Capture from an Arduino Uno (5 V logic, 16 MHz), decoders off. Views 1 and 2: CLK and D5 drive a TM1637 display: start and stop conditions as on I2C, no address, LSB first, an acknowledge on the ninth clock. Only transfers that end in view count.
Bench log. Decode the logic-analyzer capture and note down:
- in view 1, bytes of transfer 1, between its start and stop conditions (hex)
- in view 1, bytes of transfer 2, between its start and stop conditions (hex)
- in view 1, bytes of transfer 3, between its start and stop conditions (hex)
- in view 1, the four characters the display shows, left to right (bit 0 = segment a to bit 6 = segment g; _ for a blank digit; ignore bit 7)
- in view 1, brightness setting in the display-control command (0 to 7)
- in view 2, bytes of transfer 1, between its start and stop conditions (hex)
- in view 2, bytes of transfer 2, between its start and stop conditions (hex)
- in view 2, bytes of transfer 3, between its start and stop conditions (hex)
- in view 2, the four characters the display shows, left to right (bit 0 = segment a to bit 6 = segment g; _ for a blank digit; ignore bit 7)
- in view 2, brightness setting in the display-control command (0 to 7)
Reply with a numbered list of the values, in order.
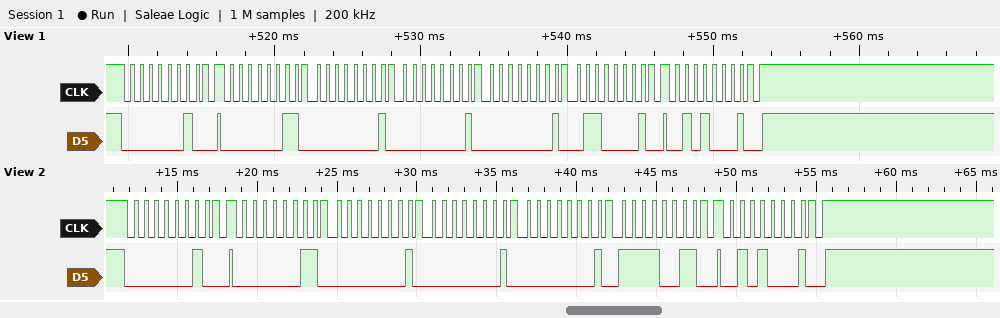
1. 40
2. C0 80 80 80 86
3. 8A
4. ___1
5. 2
6. 40
7. C0 80 80 80 CF
8. 8A
9. ___3
10. 2
